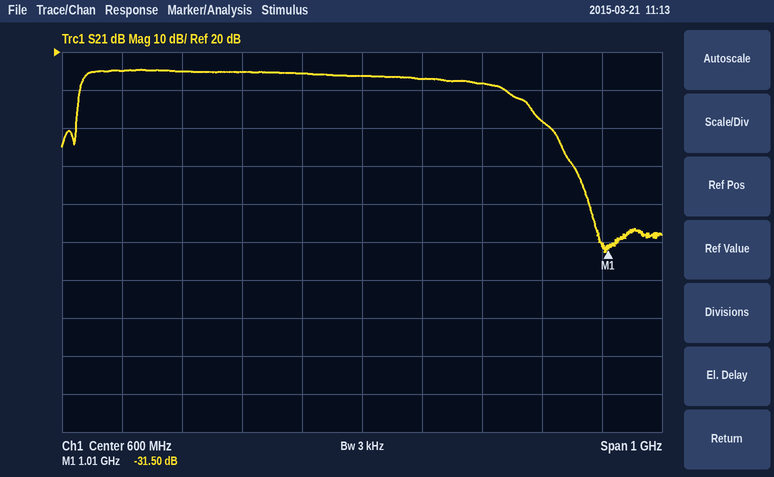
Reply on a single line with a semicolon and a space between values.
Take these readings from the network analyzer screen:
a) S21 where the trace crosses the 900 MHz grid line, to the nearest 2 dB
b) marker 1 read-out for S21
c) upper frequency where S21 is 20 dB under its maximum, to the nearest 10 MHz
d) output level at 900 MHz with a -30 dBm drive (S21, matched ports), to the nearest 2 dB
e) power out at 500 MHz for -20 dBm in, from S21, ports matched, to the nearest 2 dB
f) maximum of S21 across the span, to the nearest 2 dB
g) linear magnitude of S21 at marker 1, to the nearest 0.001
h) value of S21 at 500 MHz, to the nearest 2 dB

2 dB; -31.50 dB; 930 MHz; -28 dBm; -6 dBm; 16 dB; 0.027; 14 dB
